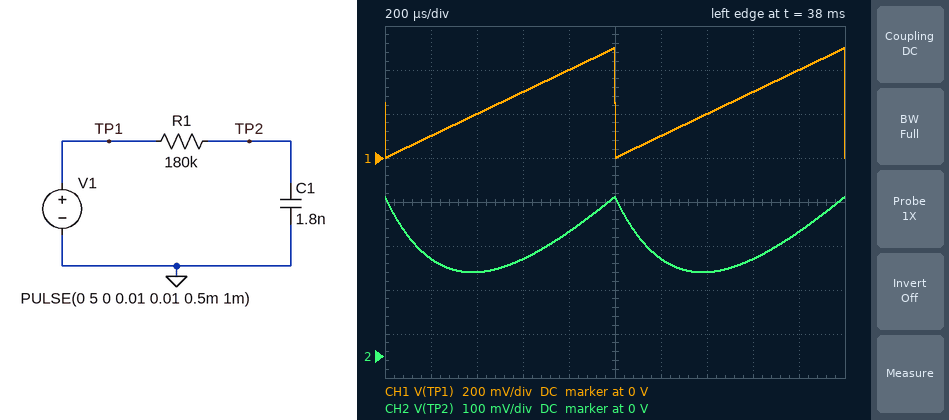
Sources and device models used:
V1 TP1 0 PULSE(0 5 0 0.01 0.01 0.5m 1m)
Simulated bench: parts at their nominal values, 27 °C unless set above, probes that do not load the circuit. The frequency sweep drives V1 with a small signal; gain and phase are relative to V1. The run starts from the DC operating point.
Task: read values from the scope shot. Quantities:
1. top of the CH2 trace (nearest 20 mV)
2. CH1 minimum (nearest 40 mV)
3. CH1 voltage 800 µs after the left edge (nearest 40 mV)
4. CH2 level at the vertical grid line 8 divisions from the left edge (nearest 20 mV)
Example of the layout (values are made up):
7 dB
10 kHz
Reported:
360 mV
0 V
400 mV
220 mV
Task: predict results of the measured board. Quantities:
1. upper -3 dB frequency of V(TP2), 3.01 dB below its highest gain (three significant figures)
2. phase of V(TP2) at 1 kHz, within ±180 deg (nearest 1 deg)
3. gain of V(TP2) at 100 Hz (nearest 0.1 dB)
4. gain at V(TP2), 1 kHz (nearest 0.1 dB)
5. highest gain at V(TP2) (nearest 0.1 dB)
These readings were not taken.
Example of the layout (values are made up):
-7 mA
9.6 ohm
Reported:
491 Hz
-64 deg
-0.2 dB
-7.1 dB
0 dB
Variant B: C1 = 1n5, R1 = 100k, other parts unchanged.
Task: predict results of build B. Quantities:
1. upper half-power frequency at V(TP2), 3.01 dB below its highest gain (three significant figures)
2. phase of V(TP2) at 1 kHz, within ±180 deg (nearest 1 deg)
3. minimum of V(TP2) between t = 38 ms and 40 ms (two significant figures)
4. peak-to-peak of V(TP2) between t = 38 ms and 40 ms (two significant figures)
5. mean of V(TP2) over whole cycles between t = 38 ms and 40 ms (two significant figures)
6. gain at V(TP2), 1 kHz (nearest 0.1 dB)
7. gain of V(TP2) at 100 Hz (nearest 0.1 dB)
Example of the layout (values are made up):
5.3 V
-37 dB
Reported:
1.06 kHz
-43 deg
140 mV
280 mV
250 mV
-2.8 dB
0 dB
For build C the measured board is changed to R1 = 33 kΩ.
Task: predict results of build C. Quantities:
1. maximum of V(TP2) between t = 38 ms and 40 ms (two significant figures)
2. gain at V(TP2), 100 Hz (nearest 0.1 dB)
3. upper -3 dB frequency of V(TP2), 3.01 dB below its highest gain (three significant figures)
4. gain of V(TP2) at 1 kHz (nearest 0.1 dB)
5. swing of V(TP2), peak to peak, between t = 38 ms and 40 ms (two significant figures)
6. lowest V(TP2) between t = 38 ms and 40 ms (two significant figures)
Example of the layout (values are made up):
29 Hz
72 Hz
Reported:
470 mV
0 dB
2.68 kHz
-0.6 dB
390 mV
84 mV
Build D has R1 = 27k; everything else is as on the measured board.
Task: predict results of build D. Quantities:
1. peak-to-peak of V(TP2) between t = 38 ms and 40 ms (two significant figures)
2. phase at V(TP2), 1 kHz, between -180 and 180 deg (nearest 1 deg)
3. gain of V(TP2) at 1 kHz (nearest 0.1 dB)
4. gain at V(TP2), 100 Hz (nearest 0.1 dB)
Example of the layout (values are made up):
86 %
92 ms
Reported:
400 mV
-17 deg
-0.4 dB
0 dB
